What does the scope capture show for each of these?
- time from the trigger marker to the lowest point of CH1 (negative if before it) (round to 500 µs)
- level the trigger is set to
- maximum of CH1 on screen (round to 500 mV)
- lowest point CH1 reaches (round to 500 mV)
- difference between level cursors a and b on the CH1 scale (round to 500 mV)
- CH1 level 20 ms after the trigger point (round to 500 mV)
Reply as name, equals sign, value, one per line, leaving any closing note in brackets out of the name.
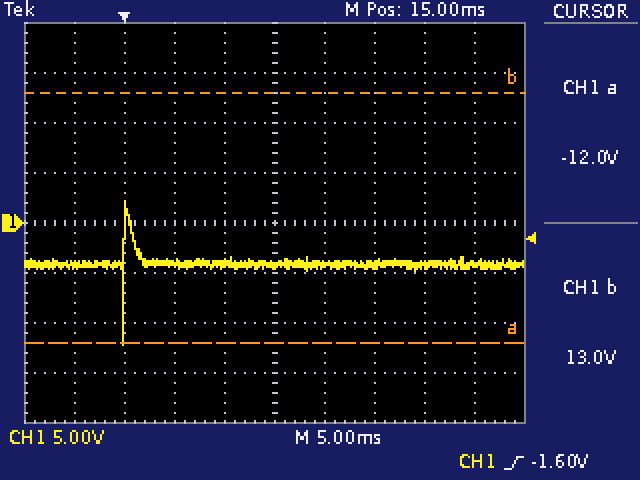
time from the trigger marker to the lowest point of CH1 (negative if before it) = 0.0 ms
level the trigger is set to = -1.60 V
maximum of CH1 on screen = 2.0 V
lowest point CH1 reaches = -12.0 V
difference between level cursors a and b on the CH1 scale = 25.0 V
CH1 level 20 ms after the trigger point = -4.0 V
